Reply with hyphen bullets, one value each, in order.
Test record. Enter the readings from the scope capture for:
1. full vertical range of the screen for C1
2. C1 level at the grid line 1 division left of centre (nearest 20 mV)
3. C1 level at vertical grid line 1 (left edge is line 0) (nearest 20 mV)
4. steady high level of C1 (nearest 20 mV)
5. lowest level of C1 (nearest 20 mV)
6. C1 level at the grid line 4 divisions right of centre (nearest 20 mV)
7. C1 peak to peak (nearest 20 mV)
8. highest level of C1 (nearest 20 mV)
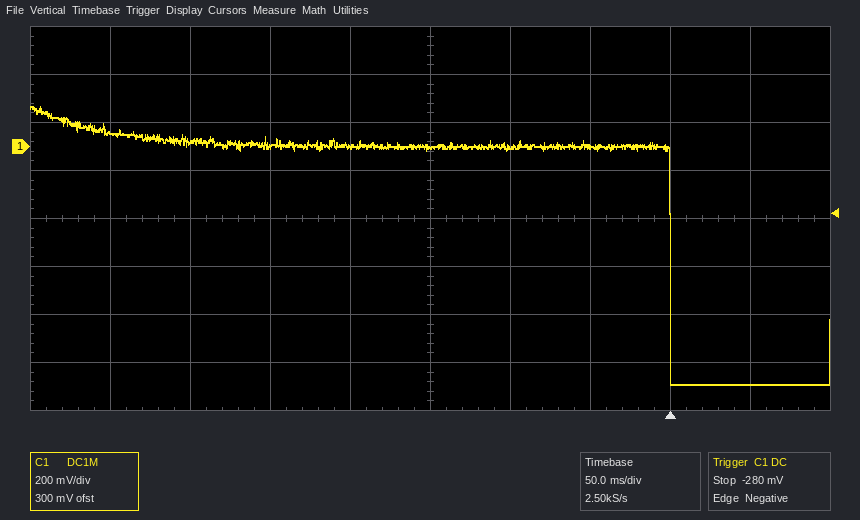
- 1.6 V
- 0 mV
- 60 mV
- 0 mV
- -1.00 V
- -1.00 V
- 1.16 V
- 160 mV
